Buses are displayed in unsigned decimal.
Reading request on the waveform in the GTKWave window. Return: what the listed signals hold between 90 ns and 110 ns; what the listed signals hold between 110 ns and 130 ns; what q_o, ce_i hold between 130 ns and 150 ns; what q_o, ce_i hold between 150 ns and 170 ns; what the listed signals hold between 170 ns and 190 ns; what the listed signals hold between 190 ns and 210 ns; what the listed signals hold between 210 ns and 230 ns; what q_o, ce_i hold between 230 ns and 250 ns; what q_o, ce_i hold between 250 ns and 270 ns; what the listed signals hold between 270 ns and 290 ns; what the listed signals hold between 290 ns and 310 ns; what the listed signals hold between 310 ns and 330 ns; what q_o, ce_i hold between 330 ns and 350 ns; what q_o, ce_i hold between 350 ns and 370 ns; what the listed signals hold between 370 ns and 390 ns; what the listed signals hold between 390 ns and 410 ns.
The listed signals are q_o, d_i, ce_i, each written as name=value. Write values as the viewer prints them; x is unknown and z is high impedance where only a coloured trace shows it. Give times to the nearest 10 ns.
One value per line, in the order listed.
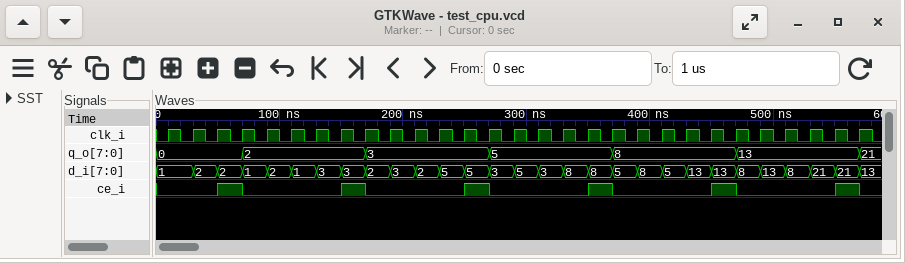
q_o=2, d_i=2, ce_i=0
q_o=2, d_i=1, ce_i=0
q_o=2, ce_i=0
q_o=2, ce_i=1
q_o=3, d_i=2, ce_i=0
q_o=3, d_i=3, ce_i=0
q_o=3, d_i=2, ce_i=0
q_o=3, ce_i=0
q_o=3, ce_i=1
q_o=5, d_i=3, ce_i=0
q_o=5, d_i=5, ce_i=0
q_o=5, d_i=3, ce_i=0
q_o=5, ce_i=0
q_o=5, ce_i=1
q_o=8, d_i=5, ce_i=0
q_o=8, d_i=8, ce_i=0
